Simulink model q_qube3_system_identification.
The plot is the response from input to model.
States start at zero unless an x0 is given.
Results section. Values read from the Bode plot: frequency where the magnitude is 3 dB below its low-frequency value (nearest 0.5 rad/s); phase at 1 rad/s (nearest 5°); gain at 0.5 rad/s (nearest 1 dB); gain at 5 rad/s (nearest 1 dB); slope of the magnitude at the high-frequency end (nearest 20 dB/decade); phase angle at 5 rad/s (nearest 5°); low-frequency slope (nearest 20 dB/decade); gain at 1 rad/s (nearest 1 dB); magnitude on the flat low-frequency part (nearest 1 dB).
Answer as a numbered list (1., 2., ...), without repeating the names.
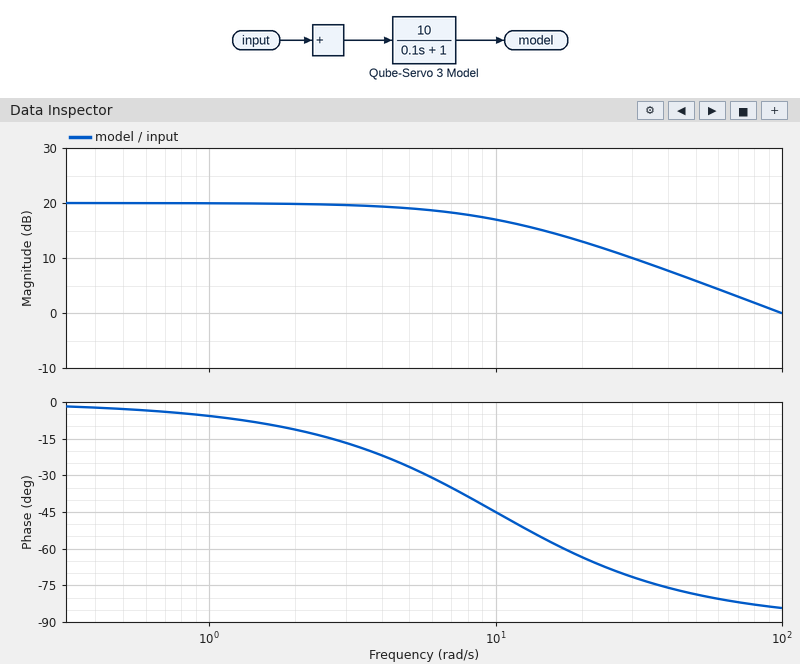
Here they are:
1. 10.0 rad/s
2. -5°
3. 20 dB
4. 19 dB
5. -20 dB/decade
6. -25°
7. 0 dB/decade
8. 20 dB
9. 20 dB
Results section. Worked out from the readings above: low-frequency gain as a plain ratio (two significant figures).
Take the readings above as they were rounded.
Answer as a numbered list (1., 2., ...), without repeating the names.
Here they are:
1. 10
